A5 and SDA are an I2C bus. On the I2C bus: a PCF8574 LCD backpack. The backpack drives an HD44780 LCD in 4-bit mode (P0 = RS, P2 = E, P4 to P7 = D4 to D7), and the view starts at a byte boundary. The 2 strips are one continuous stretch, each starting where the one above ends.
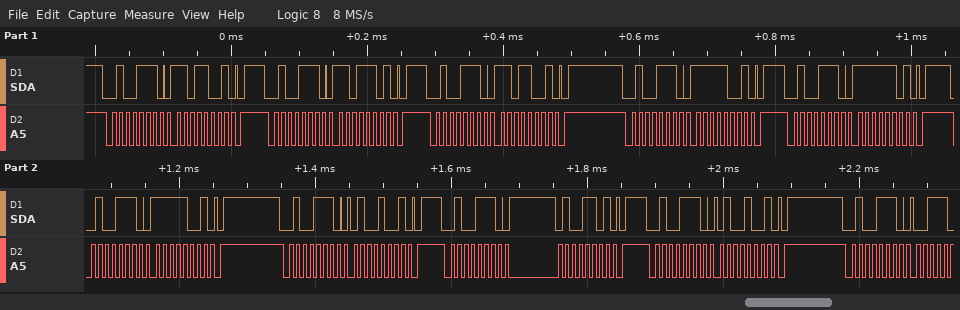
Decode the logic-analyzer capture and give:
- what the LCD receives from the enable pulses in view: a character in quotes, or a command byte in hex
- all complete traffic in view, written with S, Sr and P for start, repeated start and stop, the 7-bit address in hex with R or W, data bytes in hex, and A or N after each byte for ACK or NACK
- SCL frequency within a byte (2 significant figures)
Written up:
data 0xDF
S 27W A D9 A P S 27W A DD A P S 27W A D9 A P S 27W A F9 A P S 27W A FD A P S 27W A F9 A P S 27W A 49 A P S 27W A 4D A P S 27W A 49 A P S 27W A
100 kHz
